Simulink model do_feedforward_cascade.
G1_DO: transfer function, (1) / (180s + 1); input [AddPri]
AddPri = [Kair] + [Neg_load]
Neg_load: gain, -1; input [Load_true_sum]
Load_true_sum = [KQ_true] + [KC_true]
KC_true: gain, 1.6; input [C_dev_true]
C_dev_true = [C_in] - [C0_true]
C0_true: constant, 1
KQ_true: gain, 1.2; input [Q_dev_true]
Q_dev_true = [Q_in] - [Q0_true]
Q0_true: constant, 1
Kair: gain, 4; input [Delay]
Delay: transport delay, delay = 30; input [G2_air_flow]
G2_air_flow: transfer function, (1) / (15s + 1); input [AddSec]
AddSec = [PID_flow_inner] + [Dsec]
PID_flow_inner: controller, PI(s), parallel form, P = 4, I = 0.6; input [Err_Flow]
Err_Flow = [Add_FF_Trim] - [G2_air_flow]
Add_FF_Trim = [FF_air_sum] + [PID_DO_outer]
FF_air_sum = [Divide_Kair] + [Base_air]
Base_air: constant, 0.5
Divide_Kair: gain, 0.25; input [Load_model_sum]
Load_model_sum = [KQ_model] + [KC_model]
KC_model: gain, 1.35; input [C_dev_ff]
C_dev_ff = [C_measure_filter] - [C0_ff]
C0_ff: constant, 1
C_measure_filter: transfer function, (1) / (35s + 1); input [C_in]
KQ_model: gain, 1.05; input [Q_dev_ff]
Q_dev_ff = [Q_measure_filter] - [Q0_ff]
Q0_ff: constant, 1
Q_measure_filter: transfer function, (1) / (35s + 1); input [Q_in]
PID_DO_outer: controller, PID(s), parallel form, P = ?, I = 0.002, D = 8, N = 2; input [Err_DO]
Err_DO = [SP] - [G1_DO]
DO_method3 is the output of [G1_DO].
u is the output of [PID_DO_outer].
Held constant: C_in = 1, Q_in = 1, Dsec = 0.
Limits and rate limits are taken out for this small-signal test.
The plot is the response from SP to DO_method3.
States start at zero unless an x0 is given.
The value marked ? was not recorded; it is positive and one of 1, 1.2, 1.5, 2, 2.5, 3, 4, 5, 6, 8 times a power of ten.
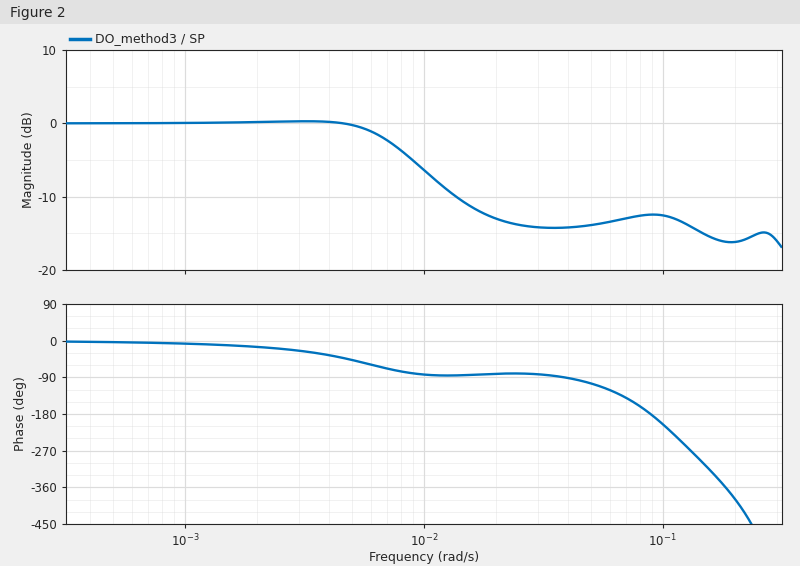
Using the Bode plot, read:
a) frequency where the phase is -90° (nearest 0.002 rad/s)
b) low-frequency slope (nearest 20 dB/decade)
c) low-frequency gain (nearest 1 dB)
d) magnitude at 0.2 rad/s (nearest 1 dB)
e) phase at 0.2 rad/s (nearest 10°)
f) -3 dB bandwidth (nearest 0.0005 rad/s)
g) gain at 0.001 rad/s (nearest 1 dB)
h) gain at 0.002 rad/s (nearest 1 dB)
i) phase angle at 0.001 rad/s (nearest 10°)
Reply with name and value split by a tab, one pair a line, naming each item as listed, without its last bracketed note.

frequency where the phase is -90°	0.038 rad/s
low-frequency slope	0 dB/decade
low-frequency gain	0 dB
magnitude at 0.2 rad/s	-16 dB
phase at 0.2 rad/s	-390°
-3 dB bandwidth	0.0075 rad/s
gain at 0.001 rad/s	0 dB
gain at 0.002 rad/s	0 dB
phase angle at 0.001 rad/s	-10°
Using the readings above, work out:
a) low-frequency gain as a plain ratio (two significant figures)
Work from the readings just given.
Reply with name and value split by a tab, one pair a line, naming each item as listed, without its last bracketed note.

low-frequency gain as a plain ratio	1.0
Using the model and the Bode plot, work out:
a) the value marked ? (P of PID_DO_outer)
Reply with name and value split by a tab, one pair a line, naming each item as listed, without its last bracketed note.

the value marked ?	0.2
